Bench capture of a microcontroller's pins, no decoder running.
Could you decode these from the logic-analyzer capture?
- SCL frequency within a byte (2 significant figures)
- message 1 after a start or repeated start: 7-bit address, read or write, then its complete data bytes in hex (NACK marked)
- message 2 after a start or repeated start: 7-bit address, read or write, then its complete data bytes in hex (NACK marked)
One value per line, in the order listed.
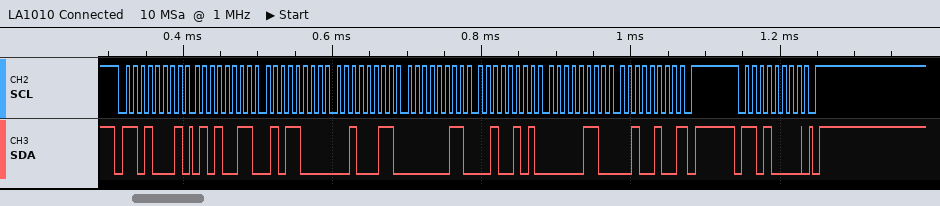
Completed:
100 kHz
0x68 read: 53 58 23 03 25 06 24 NACK
0x68 write
